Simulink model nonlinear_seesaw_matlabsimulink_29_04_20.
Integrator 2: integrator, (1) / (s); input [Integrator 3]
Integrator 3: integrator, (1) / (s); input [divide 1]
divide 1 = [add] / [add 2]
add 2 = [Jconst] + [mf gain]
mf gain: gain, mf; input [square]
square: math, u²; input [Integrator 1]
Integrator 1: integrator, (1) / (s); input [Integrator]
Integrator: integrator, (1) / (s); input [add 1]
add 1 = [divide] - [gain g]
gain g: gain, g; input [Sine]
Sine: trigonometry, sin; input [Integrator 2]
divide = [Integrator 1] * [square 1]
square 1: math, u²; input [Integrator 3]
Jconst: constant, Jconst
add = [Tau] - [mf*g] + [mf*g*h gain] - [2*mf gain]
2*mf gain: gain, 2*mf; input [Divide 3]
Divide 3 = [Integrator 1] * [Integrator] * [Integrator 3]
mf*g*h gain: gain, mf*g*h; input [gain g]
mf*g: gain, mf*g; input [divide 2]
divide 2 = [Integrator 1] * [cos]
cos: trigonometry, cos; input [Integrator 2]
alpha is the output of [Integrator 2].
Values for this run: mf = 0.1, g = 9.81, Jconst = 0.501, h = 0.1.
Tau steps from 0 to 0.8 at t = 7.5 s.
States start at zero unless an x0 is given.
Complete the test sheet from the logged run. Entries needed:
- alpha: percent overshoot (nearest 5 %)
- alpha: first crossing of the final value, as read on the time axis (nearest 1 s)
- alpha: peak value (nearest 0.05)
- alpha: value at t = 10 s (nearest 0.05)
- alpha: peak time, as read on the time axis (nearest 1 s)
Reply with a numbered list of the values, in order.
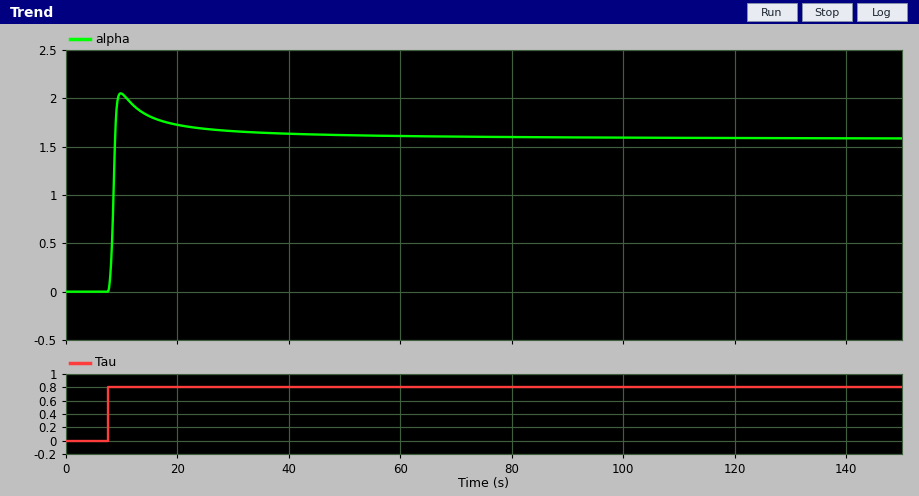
1. 30 %
2. 9 s
3. 2.05
4. 2.05
5. 10 s
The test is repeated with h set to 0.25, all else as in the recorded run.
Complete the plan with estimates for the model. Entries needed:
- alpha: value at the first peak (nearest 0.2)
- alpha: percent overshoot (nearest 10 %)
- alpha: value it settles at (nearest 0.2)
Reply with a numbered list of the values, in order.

1. 2.4
2. 50 %
3. 1.6
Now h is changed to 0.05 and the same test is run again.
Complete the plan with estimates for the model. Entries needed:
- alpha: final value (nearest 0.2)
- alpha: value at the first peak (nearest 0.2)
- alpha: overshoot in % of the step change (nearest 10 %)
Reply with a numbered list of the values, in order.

1. 1.6
2. 2.0
3. 20 %
